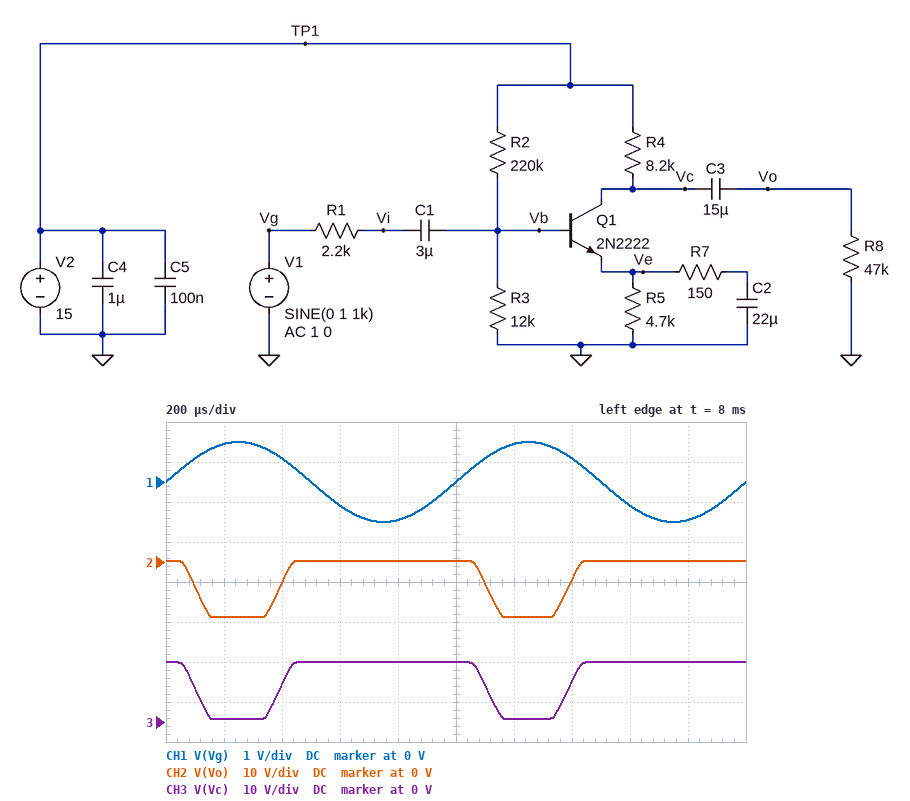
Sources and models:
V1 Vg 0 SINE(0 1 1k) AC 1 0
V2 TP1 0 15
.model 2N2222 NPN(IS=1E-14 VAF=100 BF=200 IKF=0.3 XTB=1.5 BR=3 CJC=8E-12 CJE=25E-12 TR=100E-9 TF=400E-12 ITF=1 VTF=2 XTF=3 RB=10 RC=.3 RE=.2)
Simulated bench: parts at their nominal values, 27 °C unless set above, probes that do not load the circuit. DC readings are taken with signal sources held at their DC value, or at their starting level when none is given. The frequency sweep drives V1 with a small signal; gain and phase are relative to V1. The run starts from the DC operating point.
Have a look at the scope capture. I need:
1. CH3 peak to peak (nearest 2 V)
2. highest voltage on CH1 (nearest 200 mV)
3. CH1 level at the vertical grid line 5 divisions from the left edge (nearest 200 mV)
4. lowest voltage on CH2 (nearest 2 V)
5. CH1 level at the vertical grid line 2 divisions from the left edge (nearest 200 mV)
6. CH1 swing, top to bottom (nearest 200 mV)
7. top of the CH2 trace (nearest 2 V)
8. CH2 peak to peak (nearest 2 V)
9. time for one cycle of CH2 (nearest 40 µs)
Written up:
14 V
1.0 V
0 V
-14 V
600 mV
2.0 V
0 V
14 V
1.00 ms
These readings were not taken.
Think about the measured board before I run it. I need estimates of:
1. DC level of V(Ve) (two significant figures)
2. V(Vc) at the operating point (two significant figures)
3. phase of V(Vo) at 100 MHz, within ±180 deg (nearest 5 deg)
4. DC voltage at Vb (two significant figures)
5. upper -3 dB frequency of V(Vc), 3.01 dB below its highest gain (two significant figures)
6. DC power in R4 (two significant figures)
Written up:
200 mV
15 V
-5 deg
770 mV
1.2 MHz
15 µW
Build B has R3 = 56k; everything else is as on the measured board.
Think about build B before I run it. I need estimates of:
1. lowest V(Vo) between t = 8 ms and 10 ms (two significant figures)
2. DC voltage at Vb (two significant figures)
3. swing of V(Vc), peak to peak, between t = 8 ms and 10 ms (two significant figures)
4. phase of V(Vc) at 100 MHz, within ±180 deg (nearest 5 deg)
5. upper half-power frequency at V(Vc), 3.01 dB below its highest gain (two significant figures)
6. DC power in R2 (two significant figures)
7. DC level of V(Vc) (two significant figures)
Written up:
-8.3 V
2.9 V
12 V
20 deg
520 kHz
660 µW
11 V
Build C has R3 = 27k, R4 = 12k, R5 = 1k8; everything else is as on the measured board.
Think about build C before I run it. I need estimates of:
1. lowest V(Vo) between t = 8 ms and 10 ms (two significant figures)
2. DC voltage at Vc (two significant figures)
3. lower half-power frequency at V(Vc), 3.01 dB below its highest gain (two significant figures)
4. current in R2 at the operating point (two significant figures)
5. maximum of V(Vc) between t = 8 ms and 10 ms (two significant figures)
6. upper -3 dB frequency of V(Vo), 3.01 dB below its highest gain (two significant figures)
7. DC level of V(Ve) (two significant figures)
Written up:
-7.6 V
8.7 V
35 Hz
61 µA
14 V
380 kHz
940 mV
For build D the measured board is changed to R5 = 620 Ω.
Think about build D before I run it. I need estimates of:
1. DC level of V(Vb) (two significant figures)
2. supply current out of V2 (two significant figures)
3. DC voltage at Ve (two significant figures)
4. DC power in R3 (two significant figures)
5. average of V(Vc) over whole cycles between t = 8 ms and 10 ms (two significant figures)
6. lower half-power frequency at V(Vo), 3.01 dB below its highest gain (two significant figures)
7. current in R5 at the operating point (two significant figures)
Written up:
760 mV
300 µA
150 mV
49 µW
9.6 V
27 Hz
240 µA
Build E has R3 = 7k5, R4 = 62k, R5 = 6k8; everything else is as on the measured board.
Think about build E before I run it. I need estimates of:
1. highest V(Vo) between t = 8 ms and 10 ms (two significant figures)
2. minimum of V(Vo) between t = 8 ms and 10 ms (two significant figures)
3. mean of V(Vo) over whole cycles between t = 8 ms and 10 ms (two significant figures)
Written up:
75 mV
-15 V
-5.1 V
